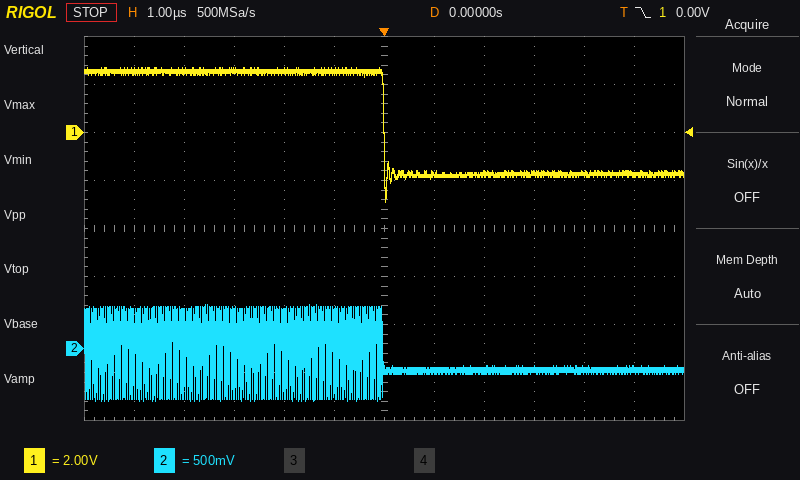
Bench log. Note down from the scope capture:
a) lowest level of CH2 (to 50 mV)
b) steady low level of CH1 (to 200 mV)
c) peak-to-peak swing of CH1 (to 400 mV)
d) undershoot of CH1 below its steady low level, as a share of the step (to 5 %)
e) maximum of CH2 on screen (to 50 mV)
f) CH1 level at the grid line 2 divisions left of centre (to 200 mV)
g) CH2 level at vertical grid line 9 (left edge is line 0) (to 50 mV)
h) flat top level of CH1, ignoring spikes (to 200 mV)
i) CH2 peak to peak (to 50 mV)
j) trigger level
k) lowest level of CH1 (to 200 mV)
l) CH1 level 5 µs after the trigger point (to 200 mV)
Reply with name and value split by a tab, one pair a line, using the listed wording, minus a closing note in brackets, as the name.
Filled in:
lowest level of CH2	-550 mV
steady low level of CH1	-1.8 V
peak-to-peak swing of CH1	5.6 V
undershoot of CH1 below its steady low level, as a share of the step	25 %
maximum of CH2 on screen	450 mV
CH1 level at the grid line 2 divisions left of centre	2.6 V
CH2 level at vertical grid line 9 (left edge is line 0)	-200 mV
flat top level of CH1, ignoring spikes	2.6 V
CH2 peak to peak	1.00 V
trigger level	0.00 V
lowest level of CH1	-2.8 V
CH1 level 5 µs after the trigger point	-1.8 V
